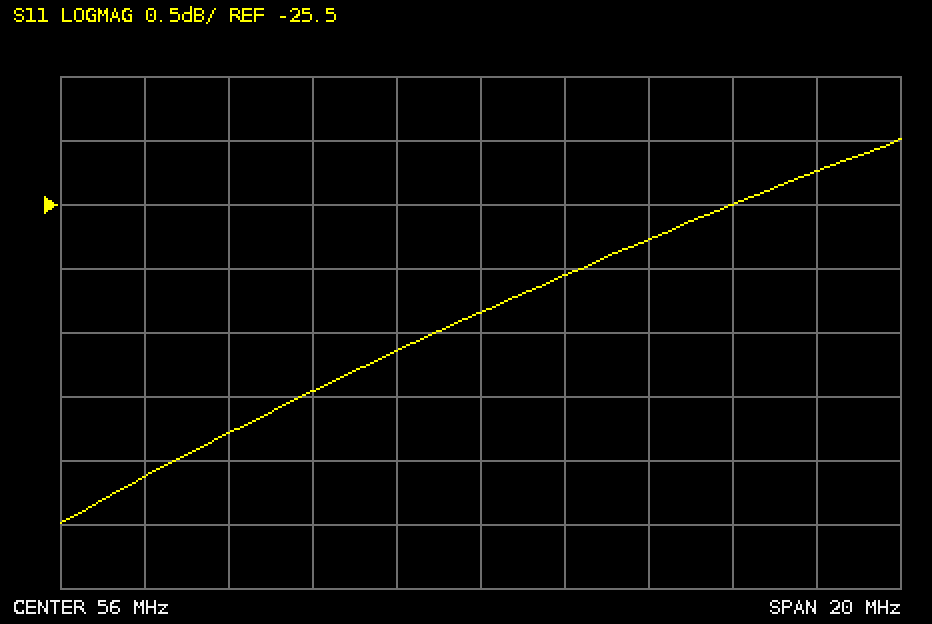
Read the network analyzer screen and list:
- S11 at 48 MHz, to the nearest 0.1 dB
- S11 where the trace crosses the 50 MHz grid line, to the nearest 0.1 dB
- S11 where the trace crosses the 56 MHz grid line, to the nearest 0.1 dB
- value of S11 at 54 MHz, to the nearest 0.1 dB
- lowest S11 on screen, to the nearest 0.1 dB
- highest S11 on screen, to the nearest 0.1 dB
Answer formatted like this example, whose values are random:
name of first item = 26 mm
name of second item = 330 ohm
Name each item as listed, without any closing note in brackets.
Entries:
S11 at 48 MHz, to the nearest 0.1 dB = -27.6 dB
S11 where the trace crosses the 50 MHz grid line, to the nearest 0.1 dB = -27.3 dB
S11 where the trace crosses the 56 MHz grid line, to the nearest 0.1 dB = -26.3 dB
value of S11 at 54 MHz, to the nearest 0.1 dB = -26.6 dB
lowest S11 on screen, to the nearest 0.1 dB = -28.0 dB
highest S11 on screen, to the nearest 0.1 dB = -25.0 dB
